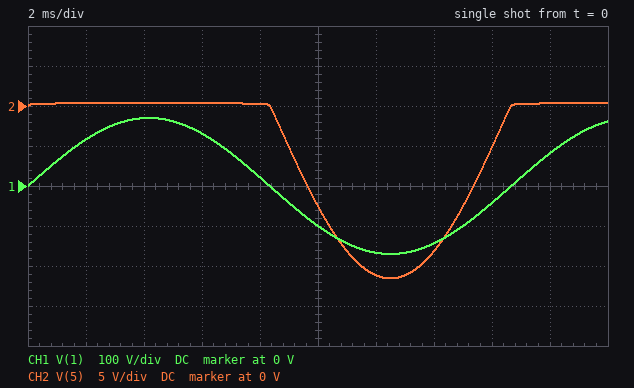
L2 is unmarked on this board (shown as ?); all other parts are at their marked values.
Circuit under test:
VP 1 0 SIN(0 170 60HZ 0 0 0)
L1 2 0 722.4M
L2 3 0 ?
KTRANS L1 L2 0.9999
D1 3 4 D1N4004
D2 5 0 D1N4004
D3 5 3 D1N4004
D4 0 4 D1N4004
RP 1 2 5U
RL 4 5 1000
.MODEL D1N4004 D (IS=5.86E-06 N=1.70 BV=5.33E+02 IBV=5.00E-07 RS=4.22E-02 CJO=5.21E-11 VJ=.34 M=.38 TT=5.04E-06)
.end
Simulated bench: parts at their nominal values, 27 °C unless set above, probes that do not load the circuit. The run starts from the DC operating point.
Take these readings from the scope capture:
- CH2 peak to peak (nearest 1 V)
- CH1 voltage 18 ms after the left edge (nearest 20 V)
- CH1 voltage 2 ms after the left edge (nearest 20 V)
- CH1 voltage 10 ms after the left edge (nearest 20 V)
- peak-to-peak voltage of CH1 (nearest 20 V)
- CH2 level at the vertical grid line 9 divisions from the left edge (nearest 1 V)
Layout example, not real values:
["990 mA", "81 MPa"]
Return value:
["22 V", "80 V", "120 V", "-100 V", "340 V", "0 V"]
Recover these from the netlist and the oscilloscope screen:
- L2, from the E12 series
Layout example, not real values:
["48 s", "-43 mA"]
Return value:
["12 mH"]
